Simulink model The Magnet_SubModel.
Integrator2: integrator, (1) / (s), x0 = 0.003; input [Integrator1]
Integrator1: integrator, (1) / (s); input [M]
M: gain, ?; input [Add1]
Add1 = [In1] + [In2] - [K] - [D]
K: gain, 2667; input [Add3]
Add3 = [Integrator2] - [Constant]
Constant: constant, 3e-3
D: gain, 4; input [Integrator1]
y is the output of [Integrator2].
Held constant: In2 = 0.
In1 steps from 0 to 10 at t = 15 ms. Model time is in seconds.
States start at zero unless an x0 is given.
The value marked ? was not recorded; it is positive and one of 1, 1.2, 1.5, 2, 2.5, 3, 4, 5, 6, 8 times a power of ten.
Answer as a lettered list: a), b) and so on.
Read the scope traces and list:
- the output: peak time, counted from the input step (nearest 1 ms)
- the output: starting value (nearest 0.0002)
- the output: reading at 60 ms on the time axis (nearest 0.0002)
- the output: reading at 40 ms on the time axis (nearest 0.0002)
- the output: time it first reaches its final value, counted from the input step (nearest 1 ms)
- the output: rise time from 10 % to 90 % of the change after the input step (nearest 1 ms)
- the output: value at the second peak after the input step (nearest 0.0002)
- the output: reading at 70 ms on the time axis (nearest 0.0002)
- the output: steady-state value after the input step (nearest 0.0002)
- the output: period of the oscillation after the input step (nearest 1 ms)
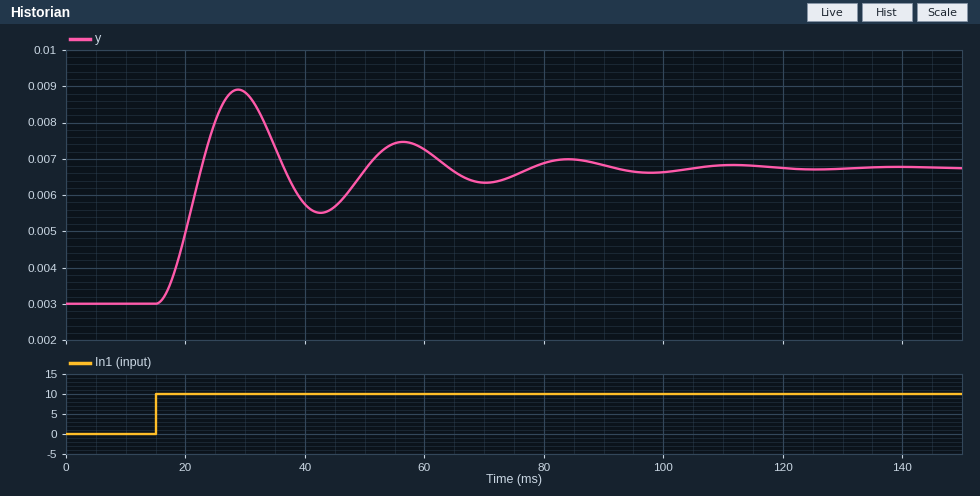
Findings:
a) 14 ms
b) 0.0030
c) 0.0072
d) 0.0058
e) 8 ms
f) 5 ms
g) 0.0074
h) 0.0064
i) 0.0068
j) 28 ms
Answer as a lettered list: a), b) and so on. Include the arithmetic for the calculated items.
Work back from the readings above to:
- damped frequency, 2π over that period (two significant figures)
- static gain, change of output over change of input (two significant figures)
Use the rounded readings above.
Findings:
a) 2π / 28 = 0.22 rad/ms
b) (0.0068 - 0.003) / (10 - 0) = 0.00038
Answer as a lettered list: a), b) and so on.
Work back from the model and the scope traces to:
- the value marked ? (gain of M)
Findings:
a) 20
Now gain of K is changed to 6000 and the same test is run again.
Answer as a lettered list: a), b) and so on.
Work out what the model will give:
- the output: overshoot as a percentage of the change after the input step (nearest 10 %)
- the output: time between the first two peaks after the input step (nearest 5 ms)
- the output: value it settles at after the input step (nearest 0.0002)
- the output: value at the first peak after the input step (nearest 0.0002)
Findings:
a) 70 %
b) 20 ms
c) 0.0046
d) 0.0058
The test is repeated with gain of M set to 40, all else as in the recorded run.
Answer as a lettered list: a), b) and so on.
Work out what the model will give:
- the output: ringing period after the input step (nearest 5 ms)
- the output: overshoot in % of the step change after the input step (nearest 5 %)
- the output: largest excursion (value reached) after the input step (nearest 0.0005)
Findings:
a) 20 ms
b) 45 %
c) 0.0085
